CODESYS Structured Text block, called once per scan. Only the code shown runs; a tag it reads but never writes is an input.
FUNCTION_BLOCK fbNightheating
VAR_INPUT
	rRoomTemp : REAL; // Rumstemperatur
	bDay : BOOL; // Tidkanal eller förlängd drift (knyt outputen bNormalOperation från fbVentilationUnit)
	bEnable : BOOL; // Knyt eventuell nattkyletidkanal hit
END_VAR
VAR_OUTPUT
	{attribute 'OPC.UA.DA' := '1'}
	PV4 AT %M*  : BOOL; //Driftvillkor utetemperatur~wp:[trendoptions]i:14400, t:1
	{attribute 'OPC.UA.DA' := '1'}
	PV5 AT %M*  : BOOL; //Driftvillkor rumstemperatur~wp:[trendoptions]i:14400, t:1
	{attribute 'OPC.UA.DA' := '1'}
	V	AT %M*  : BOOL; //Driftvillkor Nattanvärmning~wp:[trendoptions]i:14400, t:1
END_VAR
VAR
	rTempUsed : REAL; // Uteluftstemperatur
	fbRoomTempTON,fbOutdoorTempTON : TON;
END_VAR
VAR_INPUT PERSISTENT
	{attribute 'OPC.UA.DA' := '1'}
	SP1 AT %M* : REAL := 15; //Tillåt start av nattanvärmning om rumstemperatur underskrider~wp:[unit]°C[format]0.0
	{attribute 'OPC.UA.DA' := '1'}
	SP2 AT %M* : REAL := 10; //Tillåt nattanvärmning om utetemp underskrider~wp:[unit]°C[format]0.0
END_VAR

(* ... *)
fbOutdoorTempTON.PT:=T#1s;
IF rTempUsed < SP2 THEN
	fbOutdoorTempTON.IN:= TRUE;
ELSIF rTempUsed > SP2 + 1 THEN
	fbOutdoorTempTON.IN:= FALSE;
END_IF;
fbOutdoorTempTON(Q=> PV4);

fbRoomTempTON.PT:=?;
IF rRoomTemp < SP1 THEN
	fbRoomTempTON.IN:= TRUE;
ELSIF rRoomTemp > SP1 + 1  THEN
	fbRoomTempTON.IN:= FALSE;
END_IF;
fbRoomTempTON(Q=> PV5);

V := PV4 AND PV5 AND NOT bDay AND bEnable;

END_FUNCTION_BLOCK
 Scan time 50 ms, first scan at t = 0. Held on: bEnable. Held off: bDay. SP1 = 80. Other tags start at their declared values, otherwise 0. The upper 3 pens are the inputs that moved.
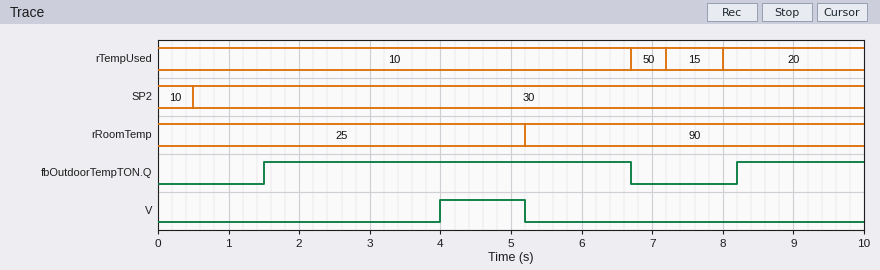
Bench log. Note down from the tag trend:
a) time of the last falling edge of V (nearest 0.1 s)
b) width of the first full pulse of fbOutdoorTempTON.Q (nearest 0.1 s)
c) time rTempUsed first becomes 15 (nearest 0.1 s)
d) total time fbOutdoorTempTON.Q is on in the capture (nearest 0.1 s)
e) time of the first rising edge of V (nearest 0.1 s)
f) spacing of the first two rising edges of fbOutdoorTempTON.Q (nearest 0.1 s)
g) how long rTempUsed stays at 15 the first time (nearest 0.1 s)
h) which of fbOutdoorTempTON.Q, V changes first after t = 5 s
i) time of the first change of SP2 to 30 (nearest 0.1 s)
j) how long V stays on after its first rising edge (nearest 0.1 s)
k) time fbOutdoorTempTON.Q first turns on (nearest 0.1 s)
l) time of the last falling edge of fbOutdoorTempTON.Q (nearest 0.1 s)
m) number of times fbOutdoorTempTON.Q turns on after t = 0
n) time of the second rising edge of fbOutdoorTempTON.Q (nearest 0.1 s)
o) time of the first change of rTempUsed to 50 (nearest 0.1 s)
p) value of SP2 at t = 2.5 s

5.2 s
5.2 s
7.2 s
7.0 s
4.0 s
6.7 s
0.8 s
V
0.5 s
1.2 s
1.5 s
6.7 s
2
8.2 s
6.7 s
30
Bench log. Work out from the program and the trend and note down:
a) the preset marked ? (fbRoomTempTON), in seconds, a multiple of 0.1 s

4.0 s
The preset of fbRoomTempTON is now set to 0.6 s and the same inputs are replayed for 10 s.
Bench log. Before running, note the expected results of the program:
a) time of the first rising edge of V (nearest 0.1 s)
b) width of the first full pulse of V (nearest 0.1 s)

1.5 s
3.7 s
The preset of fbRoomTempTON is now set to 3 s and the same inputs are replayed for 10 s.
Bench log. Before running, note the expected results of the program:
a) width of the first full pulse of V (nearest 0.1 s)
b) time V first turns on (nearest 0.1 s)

2.2 s
3.0 s
